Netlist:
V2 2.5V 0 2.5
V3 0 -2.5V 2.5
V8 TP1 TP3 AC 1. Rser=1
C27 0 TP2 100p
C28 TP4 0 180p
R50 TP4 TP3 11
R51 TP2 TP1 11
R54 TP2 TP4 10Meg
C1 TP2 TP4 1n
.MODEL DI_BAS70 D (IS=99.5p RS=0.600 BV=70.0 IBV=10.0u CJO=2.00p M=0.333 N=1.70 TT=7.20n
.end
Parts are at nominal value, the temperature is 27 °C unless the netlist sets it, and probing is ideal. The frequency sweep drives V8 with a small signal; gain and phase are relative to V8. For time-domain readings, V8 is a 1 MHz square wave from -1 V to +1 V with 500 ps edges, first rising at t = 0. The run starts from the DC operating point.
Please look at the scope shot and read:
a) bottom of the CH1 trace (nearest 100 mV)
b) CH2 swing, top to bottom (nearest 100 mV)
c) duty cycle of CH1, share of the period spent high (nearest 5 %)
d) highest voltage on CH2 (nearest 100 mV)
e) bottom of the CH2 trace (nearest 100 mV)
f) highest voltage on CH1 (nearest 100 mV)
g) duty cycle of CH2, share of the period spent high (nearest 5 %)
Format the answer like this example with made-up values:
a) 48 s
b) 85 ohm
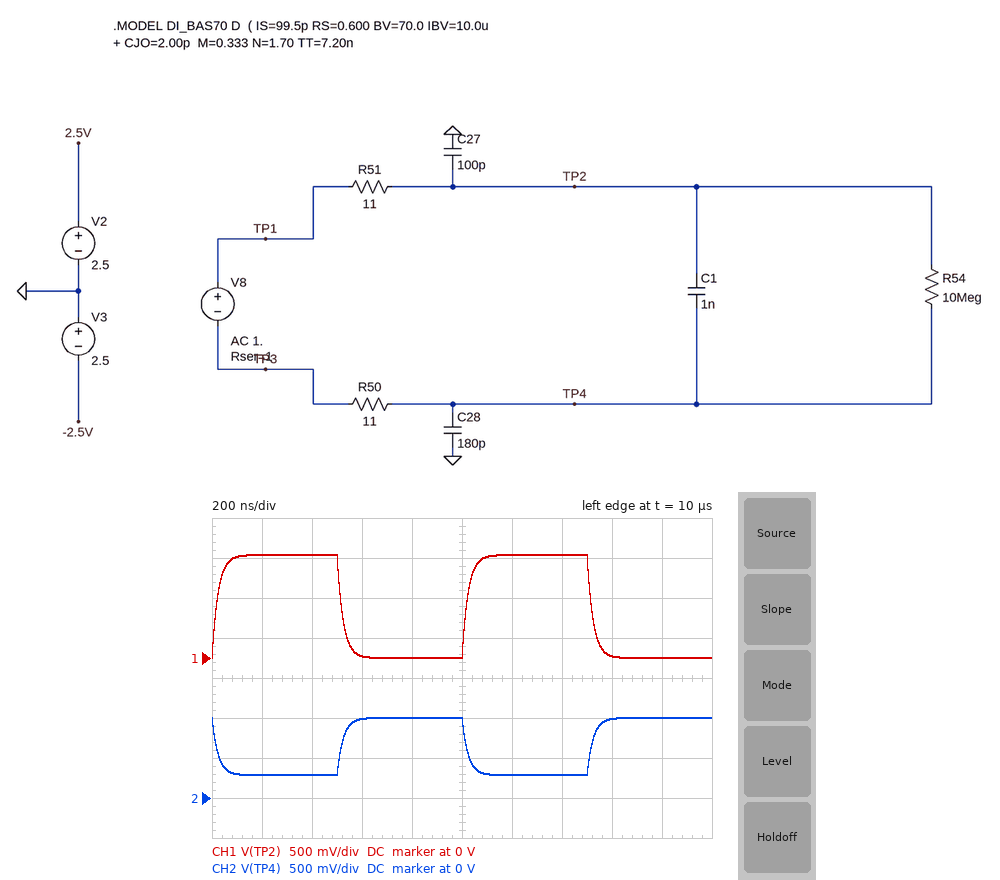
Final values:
a) 0 V
b) 700 mV
c) 50 %
d) 1.0 V
e) 300 mV
f) 1.3 V
g) 50 %
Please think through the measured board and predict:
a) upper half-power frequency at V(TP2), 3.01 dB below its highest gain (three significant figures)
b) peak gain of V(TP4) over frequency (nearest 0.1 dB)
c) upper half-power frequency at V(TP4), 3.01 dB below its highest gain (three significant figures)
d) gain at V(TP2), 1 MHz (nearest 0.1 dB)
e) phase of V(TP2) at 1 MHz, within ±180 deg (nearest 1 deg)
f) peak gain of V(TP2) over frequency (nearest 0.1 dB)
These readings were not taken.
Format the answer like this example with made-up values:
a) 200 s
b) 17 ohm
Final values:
a) 6.50 MHz
b) -8.9 dB
c) 6.50 MHz
d) -3.9 dB
e) -9 deg
f) -3.8 dB
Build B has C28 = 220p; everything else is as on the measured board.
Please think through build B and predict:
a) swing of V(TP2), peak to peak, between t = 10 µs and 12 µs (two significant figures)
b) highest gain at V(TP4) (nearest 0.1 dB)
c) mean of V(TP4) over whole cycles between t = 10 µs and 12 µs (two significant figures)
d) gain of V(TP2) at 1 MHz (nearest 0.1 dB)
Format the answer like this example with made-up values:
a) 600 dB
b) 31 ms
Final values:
a) 1.4 V
b) -10.1 dB
c) 690 mV
d) -3.4 dB
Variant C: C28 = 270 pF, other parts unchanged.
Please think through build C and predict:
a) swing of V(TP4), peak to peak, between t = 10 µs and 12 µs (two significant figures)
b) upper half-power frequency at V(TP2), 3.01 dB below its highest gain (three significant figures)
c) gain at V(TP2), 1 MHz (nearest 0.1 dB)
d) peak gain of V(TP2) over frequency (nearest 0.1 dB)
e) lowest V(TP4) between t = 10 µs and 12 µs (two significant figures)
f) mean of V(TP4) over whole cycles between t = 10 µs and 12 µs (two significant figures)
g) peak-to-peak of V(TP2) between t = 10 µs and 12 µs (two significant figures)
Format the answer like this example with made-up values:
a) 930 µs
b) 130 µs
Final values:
a) 540 mV
b) 6.45 MHz
c) -2.8 dB
d) -2.7 dB
e) 460 mV
f) 730 mV
g) 1.5 V
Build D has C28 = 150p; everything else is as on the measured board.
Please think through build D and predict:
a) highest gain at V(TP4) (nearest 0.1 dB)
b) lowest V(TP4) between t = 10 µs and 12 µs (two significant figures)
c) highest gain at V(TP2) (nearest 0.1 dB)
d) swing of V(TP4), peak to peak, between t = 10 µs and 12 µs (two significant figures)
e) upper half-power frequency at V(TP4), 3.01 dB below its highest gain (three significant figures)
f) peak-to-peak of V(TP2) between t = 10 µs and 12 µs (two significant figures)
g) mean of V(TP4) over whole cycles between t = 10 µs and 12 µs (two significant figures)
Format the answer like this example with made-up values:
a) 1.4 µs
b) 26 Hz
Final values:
a) -8.0 dB
b) 200 mV
c) -4.4 dB
d) 800 mV
e) 6.53 MHz
f) 1.2 V
g) 600 mV
